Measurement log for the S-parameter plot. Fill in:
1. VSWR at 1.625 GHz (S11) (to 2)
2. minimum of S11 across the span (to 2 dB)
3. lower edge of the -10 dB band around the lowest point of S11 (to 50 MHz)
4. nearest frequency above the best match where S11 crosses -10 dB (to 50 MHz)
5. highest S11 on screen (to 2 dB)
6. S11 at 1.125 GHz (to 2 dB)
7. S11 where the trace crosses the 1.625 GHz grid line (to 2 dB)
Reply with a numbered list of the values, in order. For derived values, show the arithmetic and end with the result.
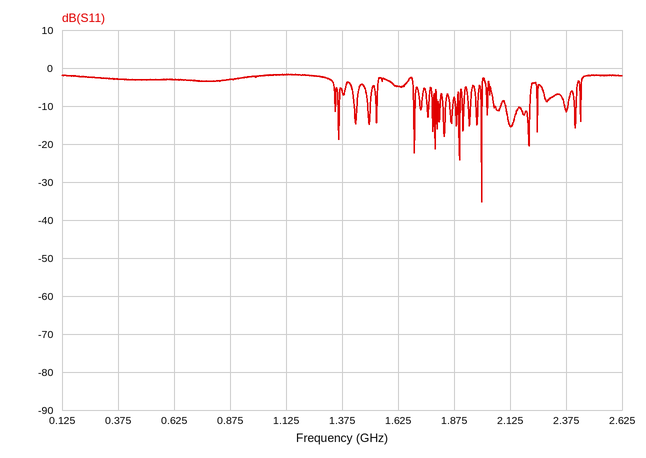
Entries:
1. |Γ| = 10^(-4/20) = 0.6310; VSWR = (1 + 0.6310)/(1 − 0.6310) ≈ 4
2. -36 dB
3. 2.00 GHz
4. 2.00 GHz
5. -2 dB
6. -2 dB
7. -4 dB
